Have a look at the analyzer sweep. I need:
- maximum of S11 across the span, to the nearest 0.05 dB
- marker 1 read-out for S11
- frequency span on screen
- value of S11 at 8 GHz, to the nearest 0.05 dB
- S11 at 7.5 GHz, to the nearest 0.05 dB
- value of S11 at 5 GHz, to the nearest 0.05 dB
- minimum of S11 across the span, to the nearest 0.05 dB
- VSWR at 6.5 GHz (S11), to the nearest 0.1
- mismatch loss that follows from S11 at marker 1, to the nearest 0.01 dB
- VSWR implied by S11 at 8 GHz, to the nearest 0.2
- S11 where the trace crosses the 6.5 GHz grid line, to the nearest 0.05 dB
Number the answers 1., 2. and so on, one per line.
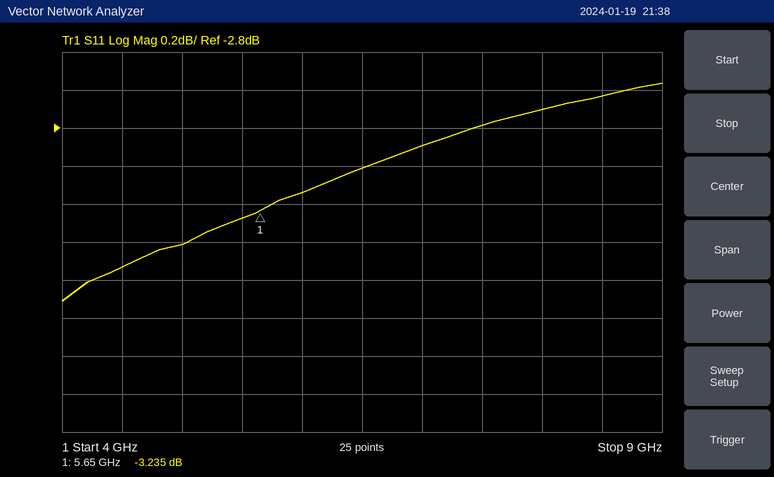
1. -2.55 dB
2. -3.235 dB
3. 5 GHz
4. -2.70 dB
5. -2.80 dB
6. -3.40 dB
7. -3.70 dB
8. 5.8
9. 2.80 dB
10. 6.4
11. -3.00 dB
